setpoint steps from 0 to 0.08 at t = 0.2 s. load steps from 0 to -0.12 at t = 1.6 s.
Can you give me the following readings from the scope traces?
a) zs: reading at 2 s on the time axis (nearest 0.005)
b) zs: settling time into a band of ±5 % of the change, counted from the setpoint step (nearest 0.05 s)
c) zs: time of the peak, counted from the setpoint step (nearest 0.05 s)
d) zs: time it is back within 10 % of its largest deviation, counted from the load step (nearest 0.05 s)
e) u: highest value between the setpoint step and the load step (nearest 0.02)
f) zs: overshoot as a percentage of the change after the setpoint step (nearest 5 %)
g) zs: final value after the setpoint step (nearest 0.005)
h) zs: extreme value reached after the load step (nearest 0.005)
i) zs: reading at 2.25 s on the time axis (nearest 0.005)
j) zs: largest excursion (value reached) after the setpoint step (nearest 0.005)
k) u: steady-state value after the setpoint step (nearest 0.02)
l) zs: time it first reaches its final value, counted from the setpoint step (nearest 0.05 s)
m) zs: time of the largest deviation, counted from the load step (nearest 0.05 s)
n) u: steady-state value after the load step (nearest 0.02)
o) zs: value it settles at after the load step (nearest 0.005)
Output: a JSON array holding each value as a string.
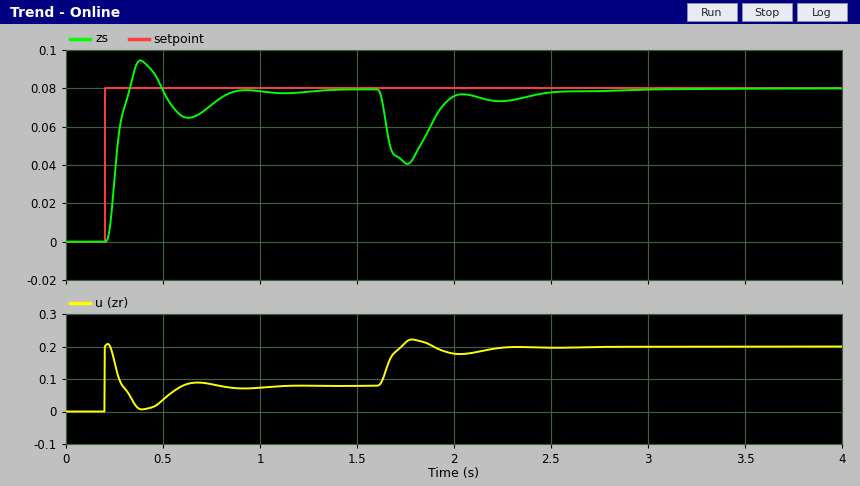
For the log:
["0.075", "0.60 s", "0.20 s", "0.80 s", "0.20", "20 %", "0.080", "0.040", "0.075", "0.095", "0.08", "0.15 s", "0.15 s", "0.20", "0.080"]
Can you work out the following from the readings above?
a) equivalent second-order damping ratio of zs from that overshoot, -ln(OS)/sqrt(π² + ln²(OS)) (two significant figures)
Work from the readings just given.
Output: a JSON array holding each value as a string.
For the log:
["0.46"]
